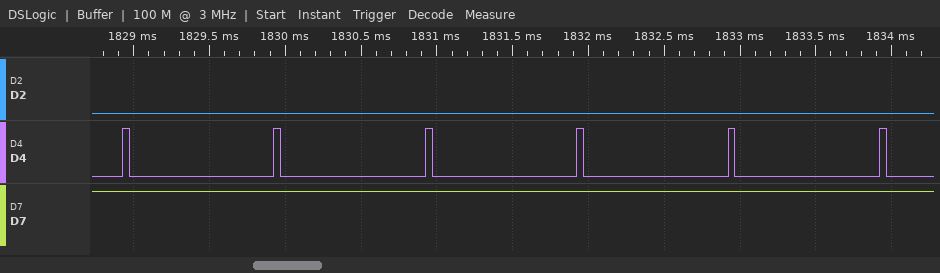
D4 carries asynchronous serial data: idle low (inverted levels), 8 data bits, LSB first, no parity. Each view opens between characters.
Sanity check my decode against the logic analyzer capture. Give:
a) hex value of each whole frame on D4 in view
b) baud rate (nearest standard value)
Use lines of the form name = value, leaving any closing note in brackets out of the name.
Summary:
hex value of each whole frame on D4 in view = FF, FF, FF, FF, FF
baud rate = 19200 baud
